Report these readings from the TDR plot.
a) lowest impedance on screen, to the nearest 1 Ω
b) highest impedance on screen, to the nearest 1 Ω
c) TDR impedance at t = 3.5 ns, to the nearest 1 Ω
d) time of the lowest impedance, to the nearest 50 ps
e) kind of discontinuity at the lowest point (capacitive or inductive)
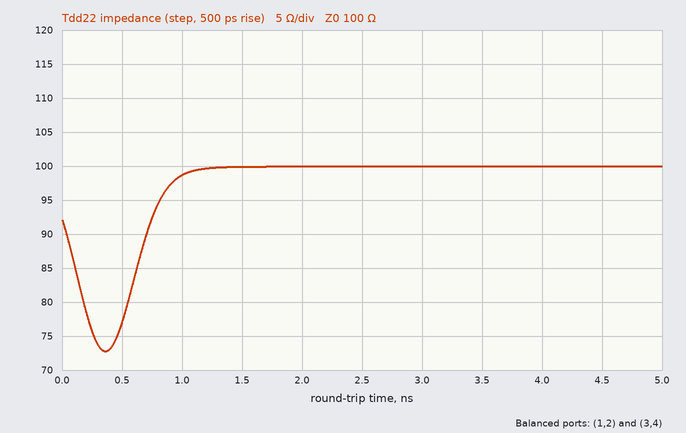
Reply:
73 Ω
100 Ω
100 Ω
350 ps
capacitive
